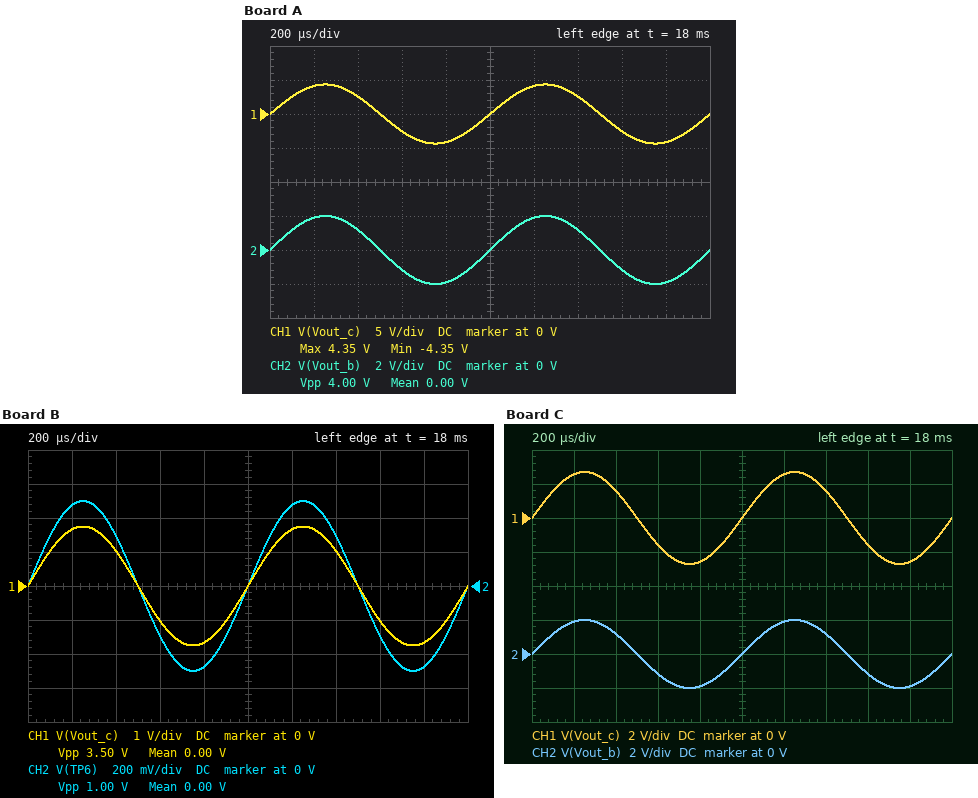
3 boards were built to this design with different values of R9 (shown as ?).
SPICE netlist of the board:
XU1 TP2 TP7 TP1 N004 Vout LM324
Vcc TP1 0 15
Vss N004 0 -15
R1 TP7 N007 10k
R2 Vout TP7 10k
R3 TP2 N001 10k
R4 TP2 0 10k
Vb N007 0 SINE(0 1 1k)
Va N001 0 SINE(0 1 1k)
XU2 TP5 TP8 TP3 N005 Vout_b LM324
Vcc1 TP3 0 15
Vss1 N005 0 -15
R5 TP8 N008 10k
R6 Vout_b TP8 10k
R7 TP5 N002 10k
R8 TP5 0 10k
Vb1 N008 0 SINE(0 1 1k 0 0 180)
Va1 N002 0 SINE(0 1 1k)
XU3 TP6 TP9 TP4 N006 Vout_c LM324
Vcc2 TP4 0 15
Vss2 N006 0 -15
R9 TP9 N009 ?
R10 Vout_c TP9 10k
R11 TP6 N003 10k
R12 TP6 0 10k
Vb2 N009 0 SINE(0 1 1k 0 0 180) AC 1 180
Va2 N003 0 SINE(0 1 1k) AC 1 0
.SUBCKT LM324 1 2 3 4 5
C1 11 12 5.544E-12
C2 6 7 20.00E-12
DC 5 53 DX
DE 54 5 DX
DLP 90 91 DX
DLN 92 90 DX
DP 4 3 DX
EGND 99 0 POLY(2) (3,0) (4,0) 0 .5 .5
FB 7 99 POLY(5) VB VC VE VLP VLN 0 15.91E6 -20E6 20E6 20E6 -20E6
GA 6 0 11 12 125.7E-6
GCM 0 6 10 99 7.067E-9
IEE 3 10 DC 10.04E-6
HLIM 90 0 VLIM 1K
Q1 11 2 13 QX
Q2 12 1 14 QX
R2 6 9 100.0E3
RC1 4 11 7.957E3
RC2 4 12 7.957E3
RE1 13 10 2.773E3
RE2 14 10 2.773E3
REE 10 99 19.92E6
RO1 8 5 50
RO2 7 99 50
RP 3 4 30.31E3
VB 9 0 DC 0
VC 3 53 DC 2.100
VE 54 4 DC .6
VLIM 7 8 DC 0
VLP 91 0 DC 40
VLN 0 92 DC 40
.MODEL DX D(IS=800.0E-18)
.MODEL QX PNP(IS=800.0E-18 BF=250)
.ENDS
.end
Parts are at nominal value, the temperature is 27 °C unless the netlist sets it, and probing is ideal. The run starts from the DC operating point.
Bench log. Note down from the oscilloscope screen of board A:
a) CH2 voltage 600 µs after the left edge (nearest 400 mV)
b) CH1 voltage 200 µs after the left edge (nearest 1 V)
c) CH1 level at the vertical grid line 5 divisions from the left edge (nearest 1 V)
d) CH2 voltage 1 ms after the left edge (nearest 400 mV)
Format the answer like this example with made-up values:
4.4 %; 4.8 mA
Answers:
-1.2 V; 4 V; 0 V; 0 V
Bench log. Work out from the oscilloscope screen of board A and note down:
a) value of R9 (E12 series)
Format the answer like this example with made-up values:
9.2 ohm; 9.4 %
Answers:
3.9 kΩ
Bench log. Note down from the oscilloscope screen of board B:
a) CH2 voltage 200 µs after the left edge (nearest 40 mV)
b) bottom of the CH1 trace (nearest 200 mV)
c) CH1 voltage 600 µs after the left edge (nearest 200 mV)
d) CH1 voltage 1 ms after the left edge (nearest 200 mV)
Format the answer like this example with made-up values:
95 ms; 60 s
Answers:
480 mV; -1.8 V; -1.0 V; 0 V
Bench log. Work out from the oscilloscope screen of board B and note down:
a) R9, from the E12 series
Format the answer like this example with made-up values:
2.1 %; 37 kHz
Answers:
12 kΩ
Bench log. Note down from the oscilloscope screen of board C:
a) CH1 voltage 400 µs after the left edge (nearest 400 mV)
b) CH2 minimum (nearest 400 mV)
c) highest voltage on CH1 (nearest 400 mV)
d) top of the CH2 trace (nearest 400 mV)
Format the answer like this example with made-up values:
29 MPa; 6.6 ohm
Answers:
1.6 V; -2.0 V; 2.8 V; 2.0 V
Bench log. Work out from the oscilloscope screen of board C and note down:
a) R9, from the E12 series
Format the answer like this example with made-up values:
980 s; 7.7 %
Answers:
6.8 kΩ
